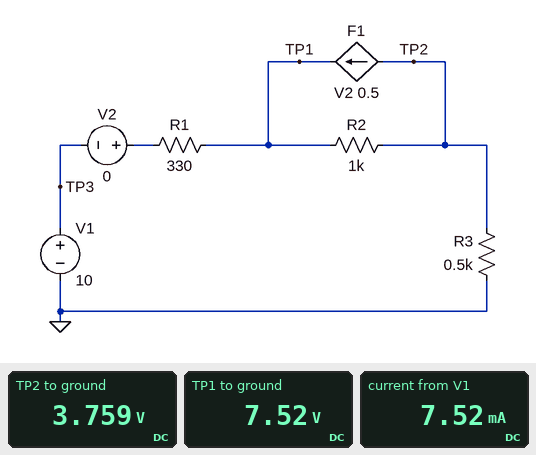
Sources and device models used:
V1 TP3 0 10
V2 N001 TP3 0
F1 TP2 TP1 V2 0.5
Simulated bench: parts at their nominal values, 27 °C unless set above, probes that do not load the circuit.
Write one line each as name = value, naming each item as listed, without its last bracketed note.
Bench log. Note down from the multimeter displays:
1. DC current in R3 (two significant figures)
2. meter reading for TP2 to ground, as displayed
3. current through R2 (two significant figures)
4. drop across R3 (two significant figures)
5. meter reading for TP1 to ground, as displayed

DC current in R3 = 7.5 mA
meter reading for TP2 to ground, as displayed = 3.759 V
current through R2 = 3.8 mA
drop across R3 = 3.8 V
meter reading for TP1 to ground, as displayed = 7.52 V
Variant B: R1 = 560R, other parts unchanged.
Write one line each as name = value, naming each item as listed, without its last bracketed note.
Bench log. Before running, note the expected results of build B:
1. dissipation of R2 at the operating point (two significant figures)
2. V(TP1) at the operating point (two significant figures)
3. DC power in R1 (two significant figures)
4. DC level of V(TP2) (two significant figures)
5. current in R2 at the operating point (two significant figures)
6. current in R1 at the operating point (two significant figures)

dissipation of R2 at the operating point = 10 mW
V(TP1) at the operating point = 6.4 V
DC power in R1 = 23 mW
DC level of V(TP2) = 3.2 V
current in R2 at the operating point = 3.2 mA
current in R1 at the operating point = 6.4 mA
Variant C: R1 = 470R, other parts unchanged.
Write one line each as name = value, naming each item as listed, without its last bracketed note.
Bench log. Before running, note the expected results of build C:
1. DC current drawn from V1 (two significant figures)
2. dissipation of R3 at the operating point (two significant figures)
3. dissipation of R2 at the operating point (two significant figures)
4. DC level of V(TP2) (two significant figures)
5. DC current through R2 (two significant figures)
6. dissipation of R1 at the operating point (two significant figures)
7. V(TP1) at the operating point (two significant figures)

DC current drawn from V1 = 6.8 mA
dissipation of R3 at the operating point = 23 mW
dissipation of R2 at the operating point = 12 mW
DC level of V(TP2) = 3.4 V
DC current through R2 = 3.4 mA
dissipation of R1 at the operating point = 22 mW
V(TP1) at the operating point = 6.8 V
